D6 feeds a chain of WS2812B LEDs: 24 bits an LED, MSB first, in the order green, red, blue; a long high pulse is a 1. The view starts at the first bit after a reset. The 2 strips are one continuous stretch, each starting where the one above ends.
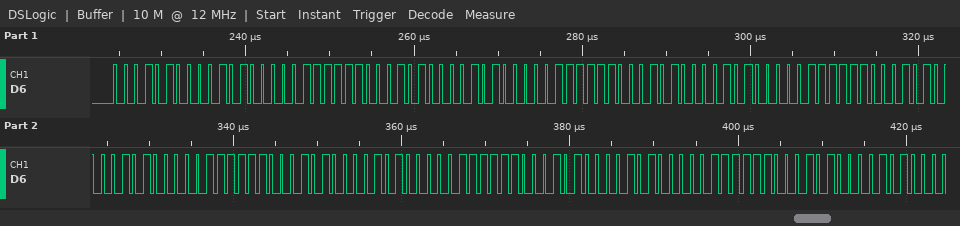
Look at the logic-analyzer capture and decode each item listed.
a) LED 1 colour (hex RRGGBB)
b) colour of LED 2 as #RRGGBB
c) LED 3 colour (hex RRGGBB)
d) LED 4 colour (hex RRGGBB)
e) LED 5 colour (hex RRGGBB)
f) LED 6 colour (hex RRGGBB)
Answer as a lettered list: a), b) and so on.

a) #28143F
b) #28143F
c) #28143F
d) #28143F
e) #28143F
f) #28143F
